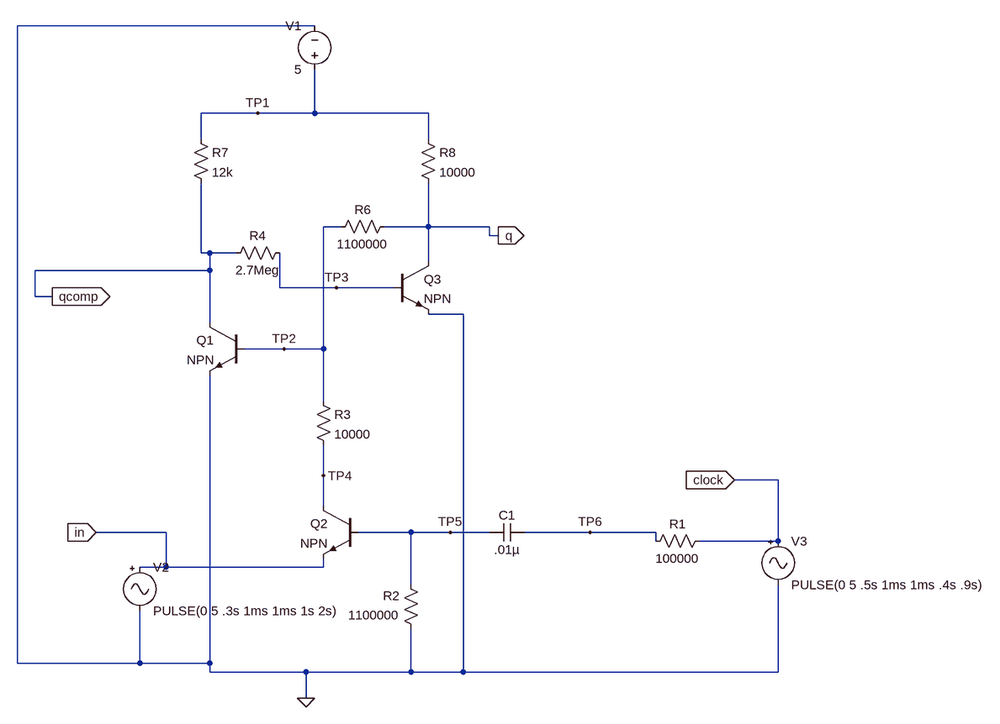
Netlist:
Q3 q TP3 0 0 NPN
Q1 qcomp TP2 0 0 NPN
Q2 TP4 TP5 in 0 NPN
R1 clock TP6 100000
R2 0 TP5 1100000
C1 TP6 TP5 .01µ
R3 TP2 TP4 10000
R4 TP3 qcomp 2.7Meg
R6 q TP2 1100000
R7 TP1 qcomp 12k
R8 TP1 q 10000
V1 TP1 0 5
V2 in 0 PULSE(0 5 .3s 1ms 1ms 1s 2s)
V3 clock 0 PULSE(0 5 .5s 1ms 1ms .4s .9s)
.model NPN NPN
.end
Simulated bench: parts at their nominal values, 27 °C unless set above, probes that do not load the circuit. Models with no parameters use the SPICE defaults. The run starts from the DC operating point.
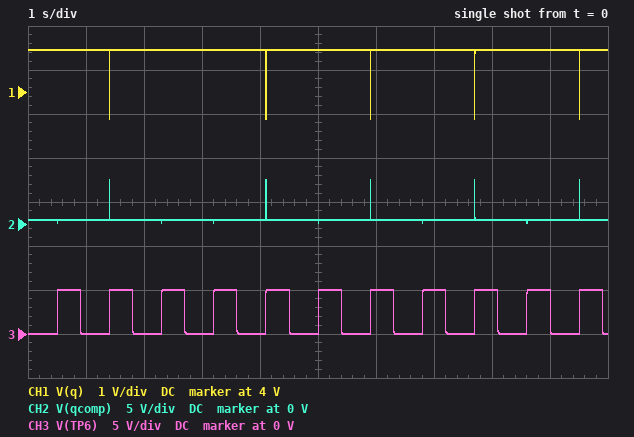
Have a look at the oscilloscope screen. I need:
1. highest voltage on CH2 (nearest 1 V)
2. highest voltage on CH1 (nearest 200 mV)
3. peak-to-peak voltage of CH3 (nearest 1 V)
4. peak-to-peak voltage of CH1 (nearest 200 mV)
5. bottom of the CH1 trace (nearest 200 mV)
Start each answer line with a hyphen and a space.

- 5 V
- 5.0 V
- 5 V
- 1.6 V
- 3.4 V
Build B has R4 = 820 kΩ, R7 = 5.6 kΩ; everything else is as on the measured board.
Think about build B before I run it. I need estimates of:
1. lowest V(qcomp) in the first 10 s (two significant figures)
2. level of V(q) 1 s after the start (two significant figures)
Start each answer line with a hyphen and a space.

- 85 mV
- 190 mV
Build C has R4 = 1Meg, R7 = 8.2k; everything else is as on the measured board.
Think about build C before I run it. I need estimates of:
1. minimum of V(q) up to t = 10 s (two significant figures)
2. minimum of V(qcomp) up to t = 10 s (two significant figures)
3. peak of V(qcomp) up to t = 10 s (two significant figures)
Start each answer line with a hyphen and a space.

- 780 mV
- 74 mV
- 5.0 V
